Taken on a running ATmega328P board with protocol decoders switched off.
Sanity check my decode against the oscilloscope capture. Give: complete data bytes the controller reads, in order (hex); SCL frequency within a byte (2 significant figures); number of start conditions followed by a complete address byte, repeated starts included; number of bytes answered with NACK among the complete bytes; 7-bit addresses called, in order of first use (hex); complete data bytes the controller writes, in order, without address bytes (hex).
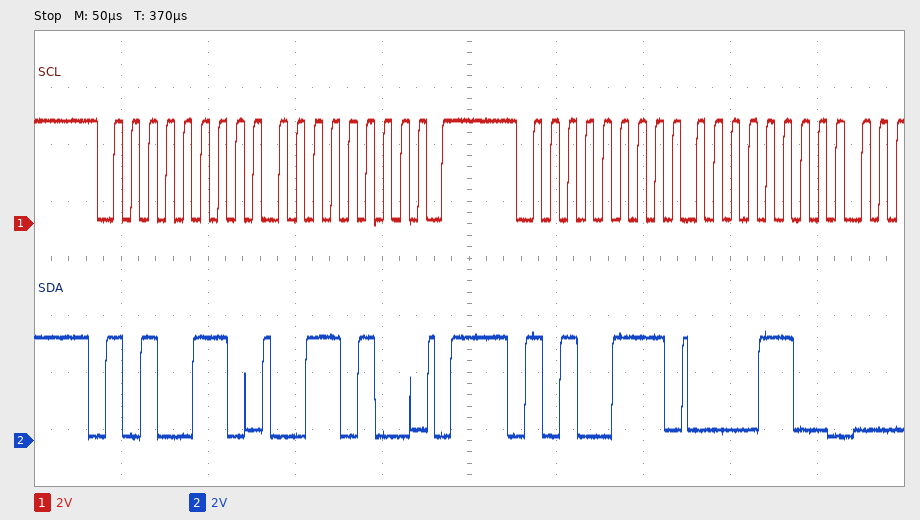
0C
100 kHz
2
0
0x53
34
